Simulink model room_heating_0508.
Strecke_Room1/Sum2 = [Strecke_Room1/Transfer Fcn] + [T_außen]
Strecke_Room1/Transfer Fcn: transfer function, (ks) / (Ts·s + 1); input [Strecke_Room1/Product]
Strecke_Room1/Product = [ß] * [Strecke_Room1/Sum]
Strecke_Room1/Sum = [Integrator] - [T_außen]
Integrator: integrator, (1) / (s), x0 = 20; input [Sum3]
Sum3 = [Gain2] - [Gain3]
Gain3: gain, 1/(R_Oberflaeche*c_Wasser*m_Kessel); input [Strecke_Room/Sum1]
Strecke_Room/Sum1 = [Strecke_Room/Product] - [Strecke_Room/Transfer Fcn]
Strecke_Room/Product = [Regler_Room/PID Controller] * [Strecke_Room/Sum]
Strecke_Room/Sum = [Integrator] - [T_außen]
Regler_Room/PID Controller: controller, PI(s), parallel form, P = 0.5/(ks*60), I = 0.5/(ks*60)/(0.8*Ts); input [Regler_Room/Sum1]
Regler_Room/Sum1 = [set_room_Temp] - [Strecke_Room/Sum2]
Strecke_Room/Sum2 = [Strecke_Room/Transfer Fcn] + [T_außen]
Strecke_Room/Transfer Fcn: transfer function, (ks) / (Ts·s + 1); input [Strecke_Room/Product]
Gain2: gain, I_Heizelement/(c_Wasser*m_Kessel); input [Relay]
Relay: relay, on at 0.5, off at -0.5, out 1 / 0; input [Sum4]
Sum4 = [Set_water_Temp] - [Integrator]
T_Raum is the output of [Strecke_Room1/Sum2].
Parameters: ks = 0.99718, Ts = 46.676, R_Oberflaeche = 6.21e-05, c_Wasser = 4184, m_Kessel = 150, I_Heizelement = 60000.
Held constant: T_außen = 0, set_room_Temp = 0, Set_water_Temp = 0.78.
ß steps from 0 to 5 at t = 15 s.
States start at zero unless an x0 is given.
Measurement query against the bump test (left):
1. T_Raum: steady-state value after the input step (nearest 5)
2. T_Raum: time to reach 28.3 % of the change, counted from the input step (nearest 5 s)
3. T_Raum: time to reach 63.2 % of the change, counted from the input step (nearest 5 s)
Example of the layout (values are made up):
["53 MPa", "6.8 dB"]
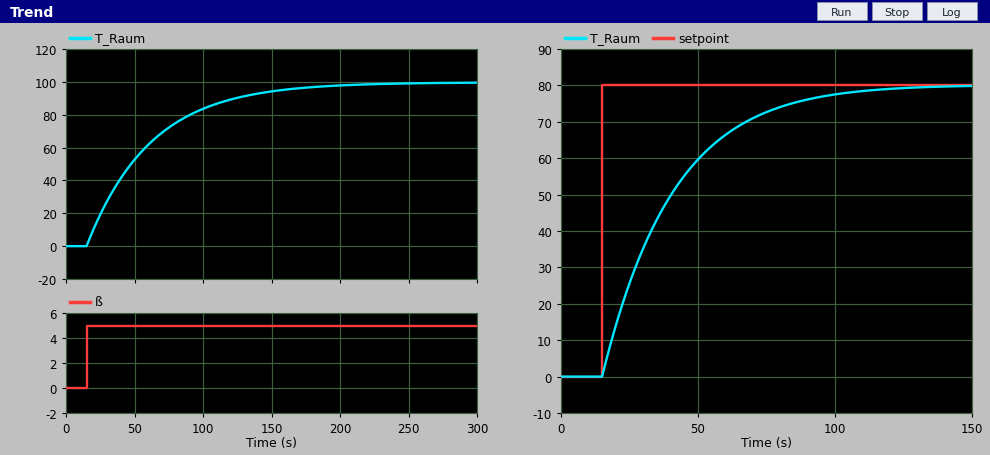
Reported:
["100", "15 s", "45 s"]
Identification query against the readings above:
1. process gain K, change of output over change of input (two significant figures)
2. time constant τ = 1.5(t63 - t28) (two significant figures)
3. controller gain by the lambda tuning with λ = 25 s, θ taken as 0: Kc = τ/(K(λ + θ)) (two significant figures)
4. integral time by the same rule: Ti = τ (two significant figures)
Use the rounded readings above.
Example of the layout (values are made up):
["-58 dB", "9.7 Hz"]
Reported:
["20", "45 s", "0.090", "45 s"]
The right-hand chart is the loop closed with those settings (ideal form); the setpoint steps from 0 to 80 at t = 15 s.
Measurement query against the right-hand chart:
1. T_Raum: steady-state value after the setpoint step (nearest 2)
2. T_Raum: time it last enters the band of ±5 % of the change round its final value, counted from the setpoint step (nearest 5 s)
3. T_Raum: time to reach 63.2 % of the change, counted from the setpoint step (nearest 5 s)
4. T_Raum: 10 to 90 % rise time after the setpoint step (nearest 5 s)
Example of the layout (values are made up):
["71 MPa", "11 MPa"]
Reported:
["80", "75 s", "25 s", "55 s"]
